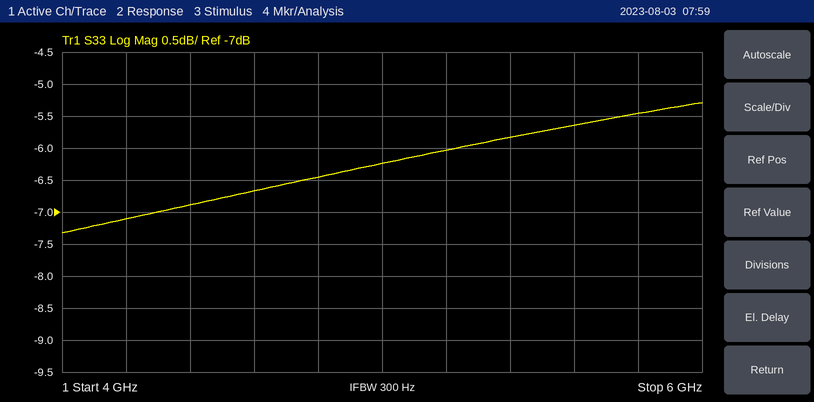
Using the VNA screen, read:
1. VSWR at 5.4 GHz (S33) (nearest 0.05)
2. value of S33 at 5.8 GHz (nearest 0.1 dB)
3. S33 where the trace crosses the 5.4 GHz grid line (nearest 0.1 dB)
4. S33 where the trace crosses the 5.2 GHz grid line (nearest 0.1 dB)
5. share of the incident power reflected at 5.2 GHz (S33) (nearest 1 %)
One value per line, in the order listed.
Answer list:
3.10
-5.5 dB
-5.8 dB
-6.0 dB
25 %
